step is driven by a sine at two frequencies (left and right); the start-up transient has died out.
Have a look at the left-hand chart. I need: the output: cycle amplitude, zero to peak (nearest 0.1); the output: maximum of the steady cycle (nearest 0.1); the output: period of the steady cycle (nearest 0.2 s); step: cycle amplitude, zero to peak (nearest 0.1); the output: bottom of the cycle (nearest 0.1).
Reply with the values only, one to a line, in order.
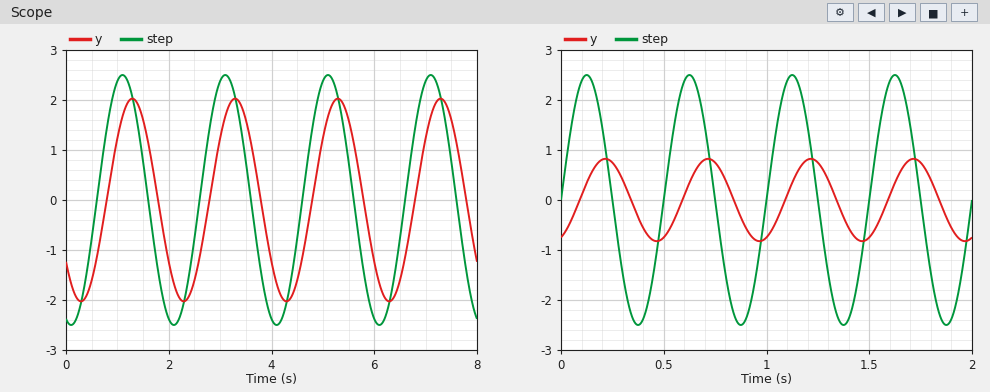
2.0
2.0
2.0 s
2.5
-2.0
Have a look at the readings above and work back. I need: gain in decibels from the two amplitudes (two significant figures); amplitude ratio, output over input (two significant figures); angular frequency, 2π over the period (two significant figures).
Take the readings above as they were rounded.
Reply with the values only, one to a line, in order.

-1.9 dB
0.80
3.1 rad/s
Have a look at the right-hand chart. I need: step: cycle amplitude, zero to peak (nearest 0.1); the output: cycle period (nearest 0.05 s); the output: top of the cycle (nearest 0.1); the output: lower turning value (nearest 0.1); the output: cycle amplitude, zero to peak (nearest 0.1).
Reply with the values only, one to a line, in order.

2.5
0.50 s
0.8
-0.8
0.8
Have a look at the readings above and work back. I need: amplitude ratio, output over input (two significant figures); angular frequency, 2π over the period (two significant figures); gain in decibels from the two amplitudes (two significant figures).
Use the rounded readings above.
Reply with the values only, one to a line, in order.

0.32
13 rad/s
-9.9 dB
